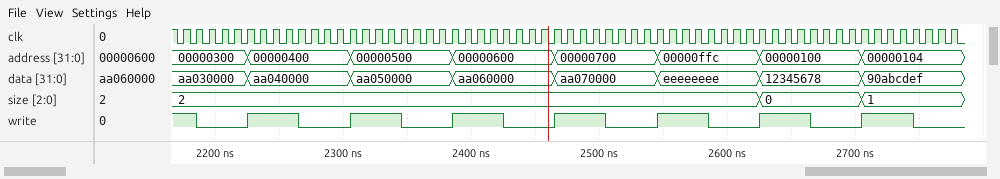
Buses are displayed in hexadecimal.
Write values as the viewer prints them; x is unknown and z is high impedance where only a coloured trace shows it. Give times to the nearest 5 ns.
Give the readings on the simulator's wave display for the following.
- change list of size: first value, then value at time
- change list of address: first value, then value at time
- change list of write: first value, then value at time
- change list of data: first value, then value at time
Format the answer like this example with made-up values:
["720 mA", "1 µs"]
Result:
["2, 0 at 2625 ns, 1 at 2705 ns", "00000300, 00000400 at 2225 ns, 00000500 at 2305 ns, 00000600 at 2385 ns, 00000700 at 2465 ns, 00000ffc at 2545 ns, 00000100 at 2625 ns, 00000104 at 2705 ns", "1, 0 at 2185 ns, 1 at 2225 ns, 0 at 2265 ns, 1 at 2305 ns, 0 at 2345 ns, 1 at 2385 ns, 0 at 2425 ns, 1 at 2465 ns, 0 at 2505 ns, 1 at 2545 ns, 0 at 2585 ns, 1 at 2625 ns, 0 at 2665 ns, 1 at 2705 ns, 0 at 2745 ns", "aa030000, aa040000 at 2225 ns, aa050000 at 2305 ns, aa060000 at 2385 ns, aa070000 at 2465 ns, eeeeeeee at 2545 ns, 12345678 at 2625 ns, 90abcdef at 2705 ns"]
